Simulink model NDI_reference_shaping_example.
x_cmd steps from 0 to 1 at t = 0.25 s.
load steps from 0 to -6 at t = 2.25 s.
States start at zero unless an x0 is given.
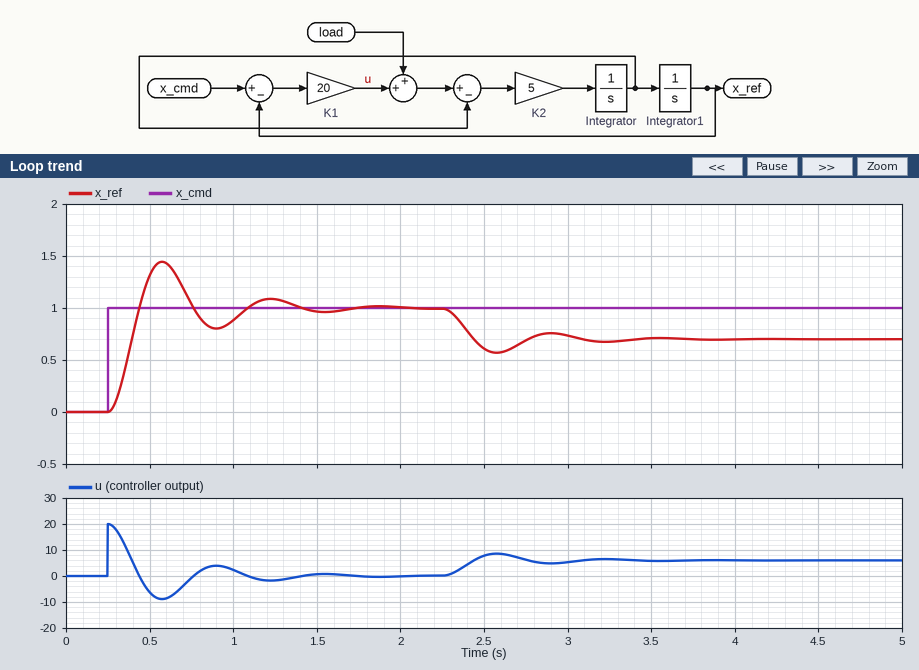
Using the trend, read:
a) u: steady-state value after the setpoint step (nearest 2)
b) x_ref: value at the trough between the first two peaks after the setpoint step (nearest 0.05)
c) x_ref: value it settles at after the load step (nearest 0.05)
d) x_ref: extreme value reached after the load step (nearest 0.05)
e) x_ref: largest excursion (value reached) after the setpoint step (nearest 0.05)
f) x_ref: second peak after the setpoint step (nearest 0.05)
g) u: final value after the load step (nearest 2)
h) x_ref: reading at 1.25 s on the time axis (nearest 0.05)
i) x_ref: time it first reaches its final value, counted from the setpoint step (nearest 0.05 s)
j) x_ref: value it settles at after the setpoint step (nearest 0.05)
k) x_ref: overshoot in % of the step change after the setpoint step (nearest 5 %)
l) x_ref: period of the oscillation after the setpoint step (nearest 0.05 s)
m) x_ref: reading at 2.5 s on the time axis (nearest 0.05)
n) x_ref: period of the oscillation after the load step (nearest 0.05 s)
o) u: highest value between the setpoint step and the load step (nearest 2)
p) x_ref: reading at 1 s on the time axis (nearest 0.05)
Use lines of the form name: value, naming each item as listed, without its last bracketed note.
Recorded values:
u: steady-state value after the setpoint step: 0
x_ref: value at the trough between the first two peaks after the setpoint step: 0.80
x_ref: value it settles at after the load step: 0.70
x_ref: extreme value reached after the load step: 0.55
x_ref: largest excursion (value reached) after the setpoint step: 1.45
x_ref: second peak after the setpoint step: 1.10
u: final value after the load step: 6
x_ref: reading at 1.25 s on the time axis: 1.10
x_ref: time it first reaches its final value, counted from the setpoint step: 0.20 s
x_ref: value it settles at after the setpoint step: 1.00
x_ref: overshoot in % of the step change after the setpoint step: 45 %
x_ref: period of the oscillation after the setpoint step: 0.65 s
x_ref: reading at 2.5 s on the time axis: 0.60
x_ref: period of the oscillation after the load step: 0.65 s
u: highest value between the setpoint step and the load step: 20
x_ref: reading at 1 s on the time axis: 0.90
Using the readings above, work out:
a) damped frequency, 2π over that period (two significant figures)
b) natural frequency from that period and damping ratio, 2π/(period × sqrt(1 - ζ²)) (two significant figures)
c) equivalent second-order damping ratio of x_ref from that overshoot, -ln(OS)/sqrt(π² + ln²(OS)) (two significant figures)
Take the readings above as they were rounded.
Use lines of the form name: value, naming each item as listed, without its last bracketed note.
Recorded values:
damped frequency, 2π over that period: 9.7 rad/s
natural frequency from that period and damping ratio, 2π/(period × sqrt(1 - ζ²)): 10.0 rad/s
equivalent second-order damping ratio of x_ref from that overshoot, -ln(OS)/sqrt(π² + ln²(OS)): 0.25
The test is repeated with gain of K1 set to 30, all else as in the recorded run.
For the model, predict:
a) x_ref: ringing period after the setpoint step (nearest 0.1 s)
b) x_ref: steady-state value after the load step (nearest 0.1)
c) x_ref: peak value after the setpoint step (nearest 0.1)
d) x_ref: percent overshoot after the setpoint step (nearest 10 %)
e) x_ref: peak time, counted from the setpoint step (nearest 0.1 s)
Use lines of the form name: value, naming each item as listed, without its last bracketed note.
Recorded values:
x_ref: ringing period after the setpoint step: 0.5 s
x_ref: steady-state value after the load step: 0.8
x_ref: peak value after the setpoint step: 1.5
x_ref: percent overshoot after the setpoint step: 50 %
x_ref: peak time, counted from the setpoint step: 0.3 s
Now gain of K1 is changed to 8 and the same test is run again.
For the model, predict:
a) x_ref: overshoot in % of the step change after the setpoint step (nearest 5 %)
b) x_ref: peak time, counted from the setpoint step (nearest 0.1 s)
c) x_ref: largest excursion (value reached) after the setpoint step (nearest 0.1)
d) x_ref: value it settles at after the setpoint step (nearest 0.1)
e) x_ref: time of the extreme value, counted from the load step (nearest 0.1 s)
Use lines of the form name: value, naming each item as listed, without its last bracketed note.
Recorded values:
x_ref: overshoot in % of the step change after the setpoint step: 25 %
x_ref: peak time, counted from the setpoint step: 0.5 s
x_ref: largest excursion (value reached) after the setpoint step: 1.3
x_ref: value it settles at after the setpoint step: 1.0
x_ref: time of the extreme value, counted from the load step: 0.5 s
